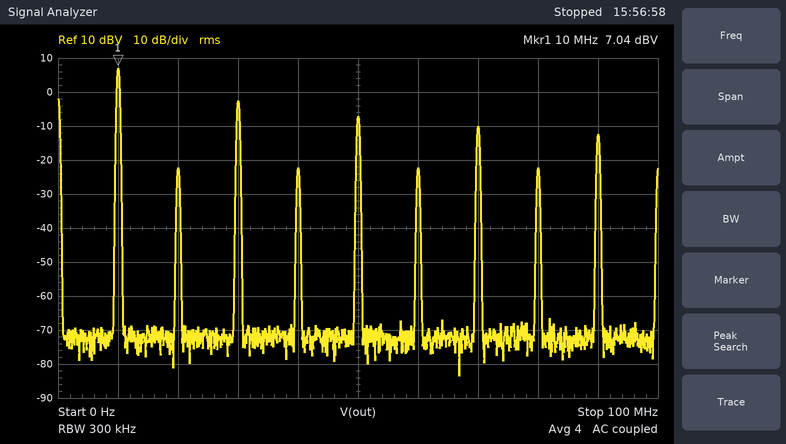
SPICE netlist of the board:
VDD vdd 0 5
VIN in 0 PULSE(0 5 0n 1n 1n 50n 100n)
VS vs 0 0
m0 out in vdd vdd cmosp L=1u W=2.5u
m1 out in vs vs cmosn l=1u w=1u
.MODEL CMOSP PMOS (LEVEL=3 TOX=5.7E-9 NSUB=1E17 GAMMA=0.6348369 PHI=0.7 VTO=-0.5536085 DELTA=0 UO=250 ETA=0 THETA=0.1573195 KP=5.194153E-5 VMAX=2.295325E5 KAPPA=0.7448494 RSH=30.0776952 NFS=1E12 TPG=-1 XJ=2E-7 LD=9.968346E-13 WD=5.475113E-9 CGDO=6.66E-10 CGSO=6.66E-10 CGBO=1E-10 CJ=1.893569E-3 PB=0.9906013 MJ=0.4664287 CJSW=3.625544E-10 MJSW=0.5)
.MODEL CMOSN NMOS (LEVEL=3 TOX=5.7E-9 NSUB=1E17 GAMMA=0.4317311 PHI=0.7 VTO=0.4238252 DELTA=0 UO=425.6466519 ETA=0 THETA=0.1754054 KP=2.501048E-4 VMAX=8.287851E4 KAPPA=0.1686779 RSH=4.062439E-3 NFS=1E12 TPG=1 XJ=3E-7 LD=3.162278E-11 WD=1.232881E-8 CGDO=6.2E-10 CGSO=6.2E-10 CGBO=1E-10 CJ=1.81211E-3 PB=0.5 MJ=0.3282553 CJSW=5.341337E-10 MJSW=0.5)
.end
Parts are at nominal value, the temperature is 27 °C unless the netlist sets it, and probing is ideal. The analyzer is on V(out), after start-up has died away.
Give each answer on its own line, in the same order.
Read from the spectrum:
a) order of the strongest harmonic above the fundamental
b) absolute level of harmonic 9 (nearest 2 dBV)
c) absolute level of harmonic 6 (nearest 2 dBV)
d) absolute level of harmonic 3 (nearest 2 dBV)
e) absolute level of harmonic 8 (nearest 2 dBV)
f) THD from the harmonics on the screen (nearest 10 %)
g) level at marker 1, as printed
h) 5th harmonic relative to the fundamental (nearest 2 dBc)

3
-12 dBV
-22 dBV
-2 dBV
-22 dBV
40 %
7.04 dBV
-14 dBc
